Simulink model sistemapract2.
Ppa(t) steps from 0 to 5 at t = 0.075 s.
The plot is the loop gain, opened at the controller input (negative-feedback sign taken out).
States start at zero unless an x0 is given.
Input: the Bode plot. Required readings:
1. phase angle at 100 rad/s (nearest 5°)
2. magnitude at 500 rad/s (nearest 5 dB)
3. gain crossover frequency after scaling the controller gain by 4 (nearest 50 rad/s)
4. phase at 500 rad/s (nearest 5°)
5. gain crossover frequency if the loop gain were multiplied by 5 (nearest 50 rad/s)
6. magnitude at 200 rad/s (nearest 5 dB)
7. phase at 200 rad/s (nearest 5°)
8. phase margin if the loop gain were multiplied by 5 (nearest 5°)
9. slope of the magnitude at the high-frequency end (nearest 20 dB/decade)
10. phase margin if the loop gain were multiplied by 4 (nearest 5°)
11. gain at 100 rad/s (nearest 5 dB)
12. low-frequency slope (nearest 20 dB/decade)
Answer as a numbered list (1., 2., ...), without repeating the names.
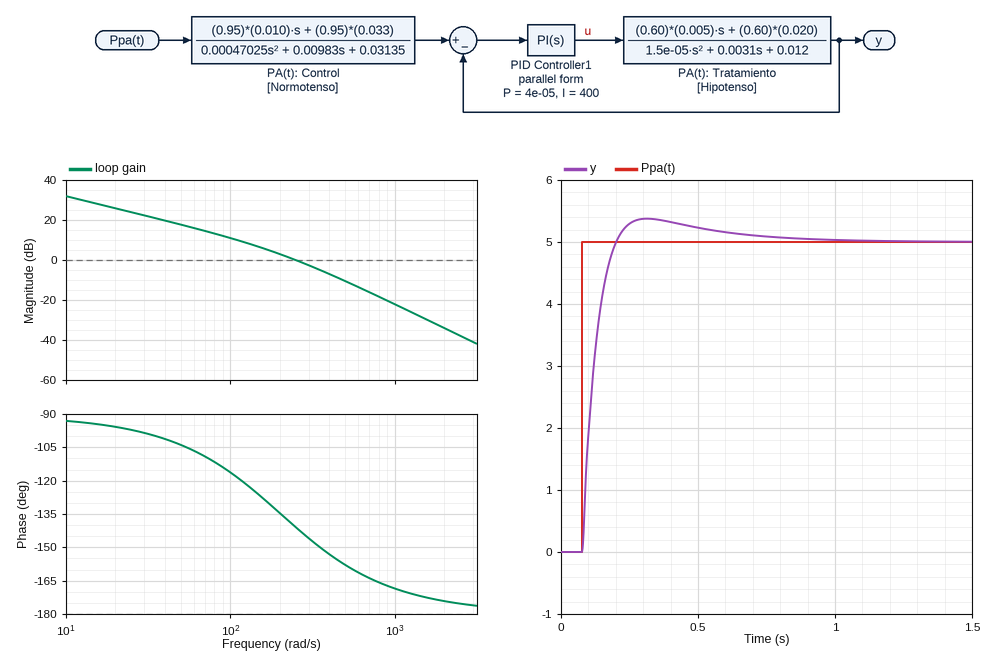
1. -115°
2. -10 dB
3. 550 rad/s
4. -160°
5. 600 rad/s
6. 5 dB
7. -135°
8. 20°
9. -40 dB/decade
10. 20°
11. 10 dB
12. -20 dB/decade
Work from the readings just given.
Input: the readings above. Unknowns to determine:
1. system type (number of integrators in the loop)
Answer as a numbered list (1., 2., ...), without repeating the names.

1. 1
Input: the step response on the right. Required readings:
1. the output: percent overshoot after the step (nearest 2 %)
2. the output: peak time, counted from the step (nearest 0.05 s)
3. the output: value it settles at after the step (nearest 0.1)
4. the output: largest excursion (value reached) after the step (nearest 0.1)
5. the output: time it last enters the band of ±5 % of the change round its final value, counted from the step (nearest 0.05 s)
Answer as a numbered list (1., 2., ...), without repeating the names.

1. 8 %
2. 0.25 s
3. 5.0
4. 5.4
5. 0.40 s
